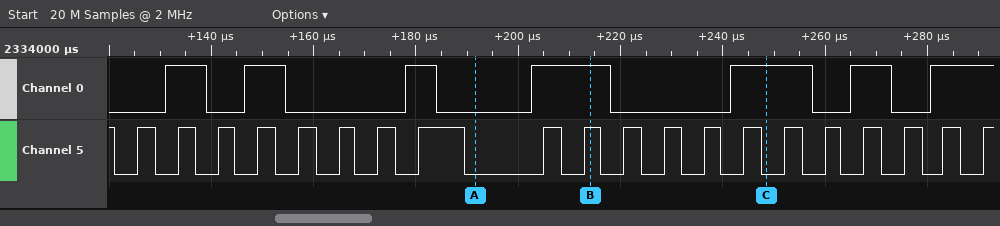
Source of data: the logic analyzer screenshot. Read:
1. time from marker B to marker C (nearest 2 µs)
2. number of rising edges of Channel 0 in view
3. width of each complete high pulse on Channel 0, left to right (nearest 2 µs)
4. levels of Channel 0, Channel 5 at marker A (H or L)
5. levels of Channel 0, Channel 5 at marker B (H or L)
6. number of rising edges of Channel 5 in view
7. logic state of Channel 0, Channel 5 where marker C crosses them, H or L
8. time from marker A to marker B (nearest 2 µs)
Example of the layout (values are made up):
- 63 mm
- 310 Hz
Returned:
- 34 µs
- 7
- 8 µs, 8 µs, 6 µs, 16 µs, 16 µs, 8 µs
- Channel 0=L, Channel 5=L
- Channel 0=H, Channel 5=H
- 20
- Channel 0=H, Channel 5=L
- 22 µs
